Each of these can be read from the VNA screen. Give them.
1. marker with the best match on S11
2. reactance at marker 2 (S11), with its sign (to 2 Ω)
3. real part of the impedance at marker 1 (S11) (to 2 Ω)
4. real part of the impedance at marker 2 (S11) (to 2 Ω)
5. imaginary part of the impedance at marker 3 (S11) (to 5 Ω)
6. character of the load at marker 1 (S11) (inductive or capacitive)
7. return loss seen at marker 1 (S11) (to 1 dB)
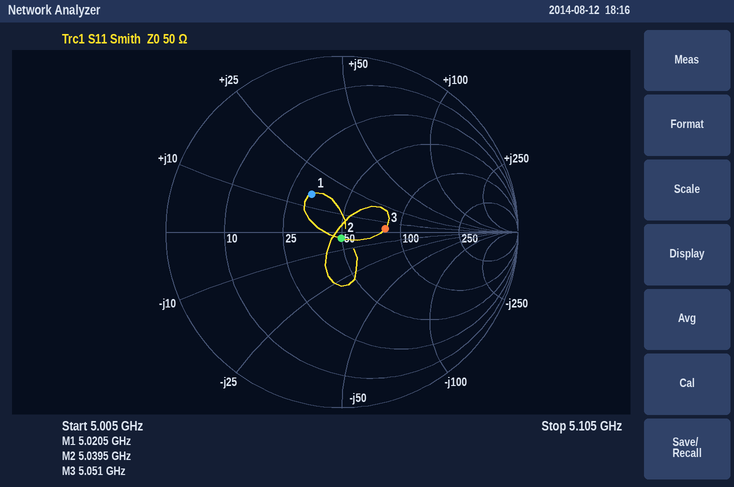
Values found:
marker 2
-4 Ω
32 Ω
50 Ω
+5 Ω
inductive
11 dB
